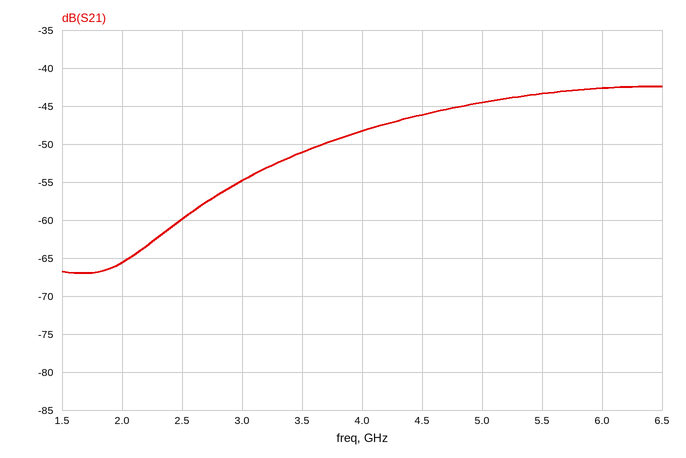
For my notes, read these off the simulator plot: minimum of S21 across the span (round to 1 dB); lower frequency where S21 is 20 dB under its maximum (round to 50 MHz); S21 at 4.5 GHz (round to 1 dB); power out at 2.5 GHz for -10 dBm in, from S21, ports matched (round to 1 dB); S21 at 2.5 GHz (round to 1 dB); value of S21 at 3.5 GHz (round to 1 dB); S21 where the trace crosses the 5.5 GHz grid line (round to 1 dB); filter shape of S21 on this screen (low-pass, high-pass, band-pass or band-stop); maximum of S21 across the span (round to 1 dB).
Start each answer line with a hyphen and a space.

- -67 dB
- 2.30 GHz
- -46 dB
- -70 dBm
- -60 dB
- -51 dB
- -43 dB
- high-pass
- -42 dB
